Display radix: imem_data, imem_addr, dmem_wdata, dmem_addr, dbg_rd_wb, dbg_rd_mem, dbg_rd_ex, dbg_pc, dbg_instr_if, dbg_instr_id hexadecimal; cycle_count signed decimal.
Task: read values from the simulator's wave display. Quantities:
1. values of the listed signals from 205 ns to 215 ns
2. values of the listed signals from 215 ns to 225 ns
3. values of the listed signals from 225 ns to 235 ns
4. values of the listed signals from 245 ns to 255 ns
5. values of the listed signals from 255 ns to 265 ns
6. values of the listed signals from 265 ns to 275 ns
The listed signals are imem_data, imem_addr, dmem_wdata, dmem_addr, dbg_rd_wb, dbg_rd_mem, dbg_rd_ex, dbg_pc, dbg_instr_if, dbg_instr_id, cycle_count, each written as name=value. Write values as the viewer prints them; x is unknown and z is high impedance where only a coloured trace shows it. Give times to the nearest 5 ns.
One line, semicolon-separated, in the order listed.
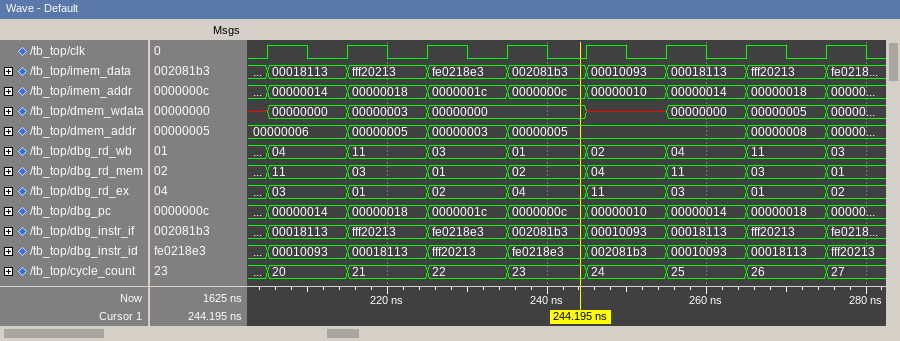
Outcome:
imem_data=00018113, imem_addr=00000014, dmem_wdata=00000000, dmem_addr=00000006, dbg_rd_wb=04, dbg_rd_mem=11, dbg_rd_ex=03, dbg_pc=00000014, dbg_instr_if=00018113, dbg_instr_id=00010093, cycle_count=20; imem_data=fff20213, imem_addr=00000018, dmem_wdata=00000003, dmem_addr=00000005, dbg_rd_wb=11, dbg_rd_mem=03, dbg_rd_ex=01, dbg_pc=00000018, dbg_instr_if=fff20213, dbg_instr_id=00018113, cycle_count=21; imem_data=fe0218e3, imem_addr=0000001c, dmem_wdata=00000000, dmem_addr=00000003, dbg_rd_wb=03, dbg_rd_mem=01, dbg_rd_ex=02, dbg_pc=0000001c, dbg_instr_if=fe0218e3, dbg_instr_id=fff20213, cycle_count=22; imem_data=00010093, imem_addr=00000010, dmem_wdata=x, dmem_addr=00000005, dbg_rd_wb=02, dbg_rd_mem=04, dbg_rd_ex=11, dbg_pc=00000010, dbg_instr_if=00010093, dbg_instr_id=002081b3, cycle_count=24; imem_data=00018113, imem_addr=00000014, dmem_wdata=00000000, dmem_addr=00000005, dbg_rd_wb=04, dbg_rd_mem=11, dbg_rd_ex=03, dbg_pc=00000014, dbg_instr_if=00018113, dbg_instr_id=00010093, cycle_count=25; imem_data=fff20213, imem_addr=00000018, dmem_wdata=00000005, dmem_addr=00000008, dbg_rd_wb=11, dbg_rd_mem=03, dbg_rd_ex=01, dbg_pc=00000018, dbg_instr_if=fff20213, dbg_instr_id=00018113, cycle_count=26
